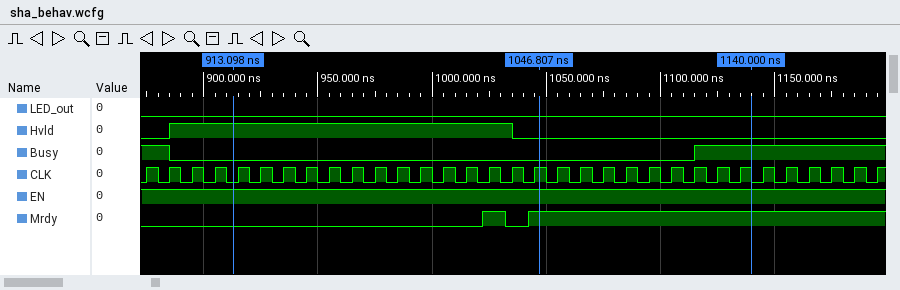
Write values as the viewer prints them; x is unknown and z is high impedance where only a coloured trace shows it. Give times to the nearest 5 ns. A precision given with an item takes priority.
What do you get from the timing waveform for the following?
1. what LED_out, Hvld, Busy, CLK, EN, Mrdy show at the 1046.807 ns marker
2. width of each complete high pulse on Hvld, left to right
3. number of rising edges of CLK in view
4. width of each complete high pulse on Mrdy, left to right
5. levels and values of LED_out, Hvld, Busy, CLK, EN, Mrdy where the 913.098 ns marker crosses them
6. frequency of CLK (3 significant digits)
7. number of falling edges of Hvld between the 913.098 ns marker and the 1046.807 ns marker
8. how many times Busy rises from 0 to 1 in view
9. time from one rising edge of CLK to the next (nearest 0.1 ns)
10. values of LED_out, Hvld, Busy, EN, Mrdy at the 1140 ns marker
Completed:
LED_out=0, Hvld=0, Busy=0, CLK=1, EN=1, Mrdy=1
150 ns
33
10 ns
LED_out=0, Hvld=1, Busy=0, CLK=0, EN=1, Mrdy=0
100 MHz
1
1
10 ns
LED_out=0, Hvld=0, Busy=1, EN=1, Mrdy=1
